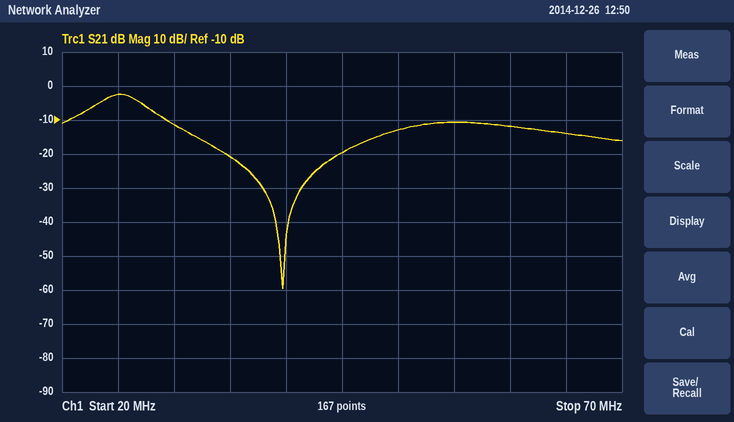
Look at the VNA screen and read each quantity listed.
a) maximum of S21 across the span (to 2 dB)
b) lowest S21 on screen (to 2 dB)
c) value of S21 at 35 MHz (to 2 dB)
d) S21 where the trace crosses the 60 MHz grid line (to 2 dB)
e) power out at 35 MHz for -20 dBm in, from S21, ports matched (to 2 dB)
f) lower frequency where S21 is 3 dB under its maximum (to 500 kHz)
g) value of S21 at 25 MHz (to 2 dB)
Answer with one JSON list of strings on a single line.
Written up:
["-2 dB", "-60 dB", "-20 dB", "-12 dB", "-40 dBm", "23.0 MHz", "-2 dB"]
